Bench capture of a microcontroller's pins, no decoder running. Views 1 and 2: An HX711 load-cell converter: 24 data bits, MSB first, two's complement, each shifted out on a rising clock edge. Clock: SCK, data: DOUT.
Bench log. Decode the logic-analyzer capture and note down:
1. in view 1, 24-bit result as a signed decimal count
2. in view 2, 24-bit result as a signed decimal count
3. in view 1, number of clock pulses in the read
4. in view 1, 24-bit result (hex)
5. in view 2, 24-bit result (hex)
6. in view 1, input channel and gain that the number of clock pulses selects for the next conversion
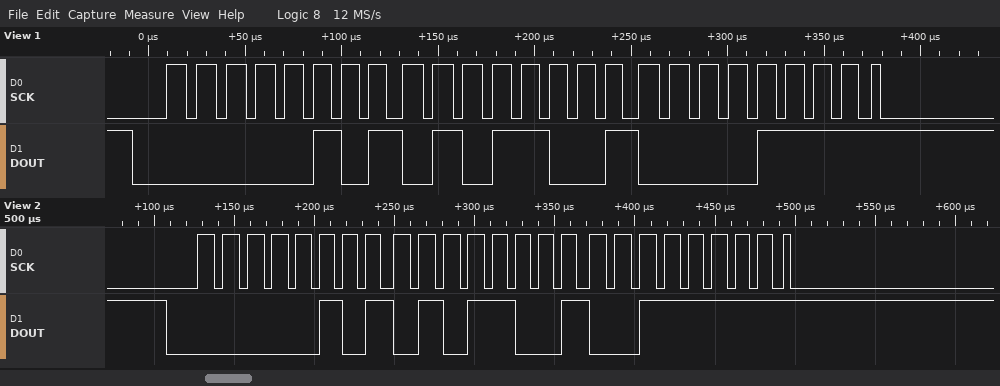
350479
350527
25
0x05590F
0x05593F
channel A, gain 128
